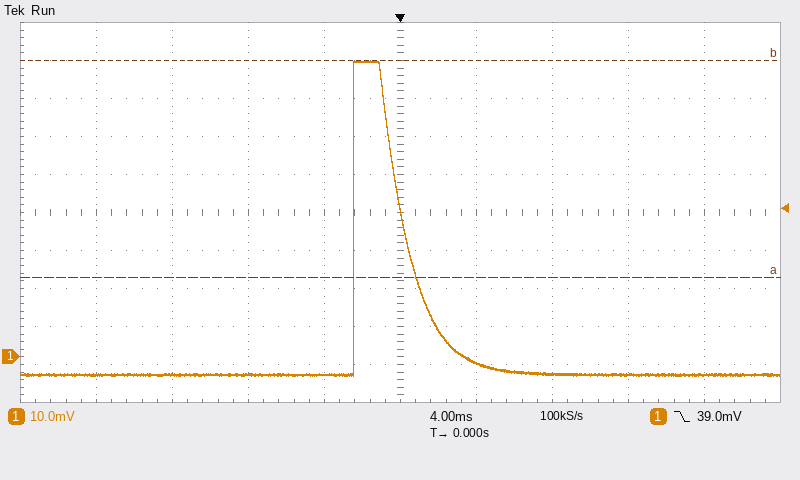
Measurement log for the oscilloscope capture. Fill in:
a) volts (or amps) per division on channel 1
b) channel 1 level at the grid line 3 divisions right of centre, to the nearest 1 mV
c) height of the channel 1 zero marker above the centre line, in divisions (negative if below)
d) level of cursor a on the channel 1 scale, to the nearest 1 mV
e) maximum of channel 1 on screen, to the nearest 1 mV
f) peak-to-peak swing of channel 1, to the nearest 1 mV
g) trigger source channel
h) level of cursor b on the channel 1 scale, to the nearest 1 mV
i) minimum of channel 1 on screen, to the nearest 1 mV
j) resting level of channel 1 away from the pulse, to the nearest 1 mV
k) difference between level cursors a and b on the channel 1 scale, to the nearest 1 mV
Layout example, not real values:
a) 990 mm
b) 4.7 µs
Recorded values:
a) 10 mV
b) -5 mV
c) -3.8 div
d) 21 mV
e) 78 mV
f) 83 mV
g) channel 1
h) 78 mV
i) -5 mV
j) -5 mV
k) 57 mV
